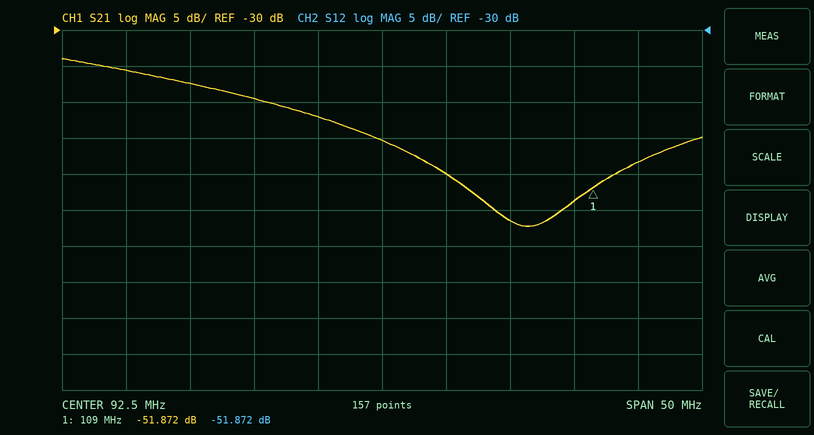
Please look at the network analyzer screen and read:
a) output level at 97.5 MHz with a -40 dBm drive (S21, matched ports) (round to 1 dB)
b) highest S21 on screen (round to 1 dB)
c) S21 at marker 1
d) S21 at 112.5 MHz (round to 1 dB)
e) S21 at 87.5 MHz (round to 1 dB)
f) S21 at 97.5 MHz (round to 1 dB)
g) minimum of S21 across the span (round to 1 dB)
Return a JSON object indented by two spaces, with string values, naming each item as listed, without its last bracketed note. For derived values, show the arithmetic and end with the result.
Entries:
{
  "output level at 97.5 MHz with a -40 dBm drive (S21, matched ports)": "-40 dBm + (-50 dB) = -90 dBm",
  "highest S21 on screen": "-34 dB",
  "S21 at marker 1": "-51.872 dB",
  "S21 at 112.5 MHz": "-48 dB",
  "S21 at 87.5 MHz": "-42 dB",
  "S21 at 97.5 MHz": "-50 dB",
  "minimum of S21 across the span": "-57 dB"
}
